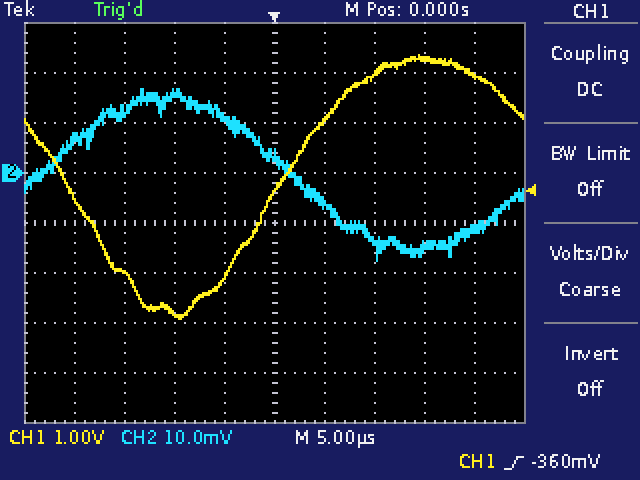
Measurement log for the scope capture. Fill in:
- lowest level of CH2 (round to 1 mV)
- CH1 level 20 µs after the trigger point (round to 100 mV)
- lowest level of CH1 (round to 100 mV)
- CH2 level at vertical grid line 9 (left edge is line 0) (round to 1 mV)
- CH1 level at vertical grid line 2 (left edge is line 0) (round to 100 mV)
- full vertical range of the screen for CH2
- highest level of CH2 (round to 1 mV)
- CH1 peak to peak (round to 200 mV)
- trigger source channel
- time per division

-18 mV
1.9 V
-2.9 V
-11 mV
-2.0 V
80 mV
17 mV
5.2 V
CH1
5 µs
